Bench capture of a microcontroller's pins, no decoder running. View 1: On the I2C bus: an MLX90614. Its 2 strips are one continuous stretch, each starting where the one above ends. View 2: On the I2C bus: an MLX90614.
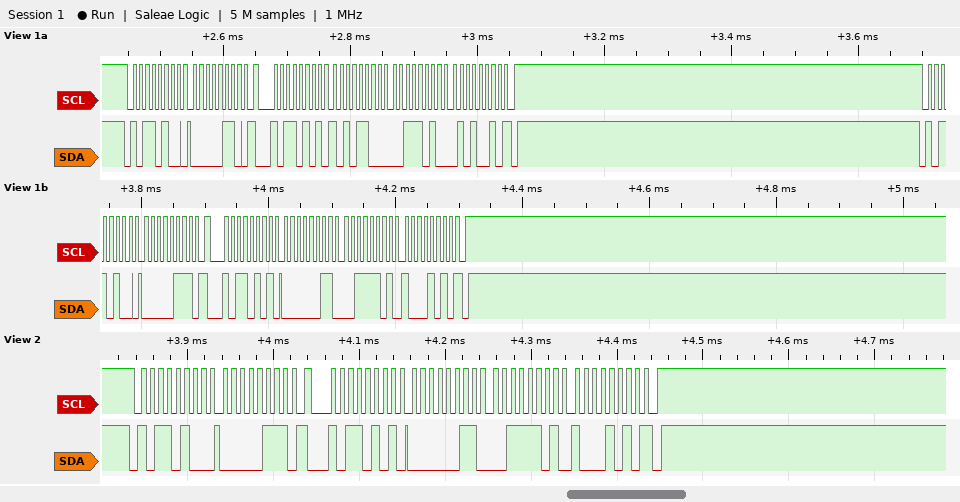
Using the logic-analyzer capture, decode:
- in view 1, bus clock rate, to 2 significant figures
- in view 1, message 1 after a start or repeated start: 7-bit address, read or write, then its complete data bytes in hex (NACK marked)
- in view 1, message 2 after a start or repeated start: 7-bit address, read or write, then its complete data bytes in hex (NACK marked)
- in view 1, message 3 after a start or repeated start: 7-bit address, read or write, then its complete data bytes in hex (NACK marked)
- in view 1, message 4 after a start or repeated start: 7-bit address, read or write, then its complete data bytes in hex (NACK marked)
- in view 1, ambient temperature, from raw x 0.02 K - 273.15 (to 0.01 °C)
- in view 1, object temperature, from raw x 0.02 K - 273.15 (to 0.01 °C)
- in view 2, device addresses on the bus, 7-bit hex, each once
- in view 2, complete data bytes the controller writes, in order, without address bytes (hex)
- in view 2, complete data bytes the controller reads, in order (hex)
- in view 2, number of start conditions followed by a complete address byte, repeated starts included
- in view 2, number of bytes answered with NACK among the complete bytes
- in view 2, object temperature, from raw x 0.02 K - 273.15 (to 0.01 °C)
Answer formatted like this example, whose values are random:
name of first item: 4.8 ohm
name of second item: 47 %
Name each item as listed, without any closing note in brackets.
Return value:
in view 1, bus clock rate, to 2 significant figures: 100 kHz
in view 1, message 1 after a start or repeated start: 7-bit address, read or write, then its complete data bytes in hex: 0x5A write: 06
in view 1, message 2 after a start or repeated start: 7-bit address, read or write, then its complete data bytes in hex: 0x5A read: AC 3A 52 NACK
in view 1, message 3 after a start or repeated start: 7-bit address, read or write, then its complete data bytes in hex: 0x5A write: 07
in view 1, message 4 after a start or repeated start: 7-bit address, read or write, then its complete data bytes in hex: 0x5A read: 03 3D 8A NACK
in view 1, ambient temperature, from raw x 0.02 K - 273.15: 27.25 °C
in view 1, object temperature, from raw x 0.02 K - 273.15: 39.23 °C
in view 2, device addresses on the bus, 7-bit hex, each once: 0x5A
in view 2, complete data bytes the controller writes, in order, without address bytes: 07
in view 2, complete data bytes the controller reads, in order: 03 3D 8A
in view 2, number of start conditions followed by a complete address byte, repeated starts included: 2
in view 2, number of bytes answered with NACK among the complete bytes: 1
in view 2, object temperature, from raw x 0.02 K - 273.15: 39.23 °C
